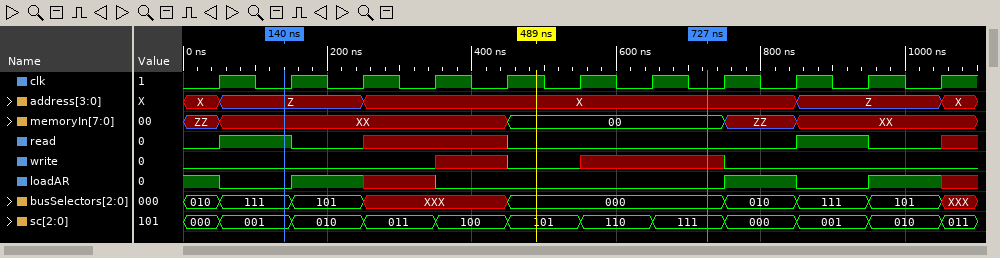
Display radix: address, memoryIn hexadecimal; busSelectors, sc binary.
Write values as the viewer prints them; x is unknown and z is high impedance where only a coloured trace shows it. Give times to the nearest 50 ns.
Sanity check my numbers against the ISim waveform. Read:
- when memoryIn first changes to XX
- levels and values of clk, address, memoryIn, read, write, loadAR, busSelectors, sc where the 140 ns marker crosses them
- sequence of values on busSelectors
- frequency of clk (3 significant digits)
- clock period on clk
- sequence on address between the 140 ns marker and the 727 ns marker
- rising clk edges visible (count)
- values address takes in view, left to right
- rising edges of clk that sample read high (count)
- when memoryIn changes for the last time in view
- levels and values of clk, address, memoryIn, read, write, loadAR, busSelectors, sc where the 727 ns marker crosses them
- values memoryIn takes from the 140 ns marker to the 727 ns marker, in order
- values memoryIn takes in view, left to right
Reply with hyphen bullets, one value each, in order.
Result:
- 50 ns
- clk=0, address=Z, memoryIn=XX, read=1, write=0, loadAR=0, busSelectors=111, sc=001
- 010, 111, 101, XXX, 000, 010, 111, 101, XXX
- 10.0 MHz
- 100 ns
- Z, X
- 11
- X, Z, X, Z, X
- 2
- 850 ns
- clk=0, address=X, memoryIn=00, read=0, write=x, loadAR=0, busSelectors=000, sc=111
- XX, 00
- ZZ, XX, 00, ZZ, XX
